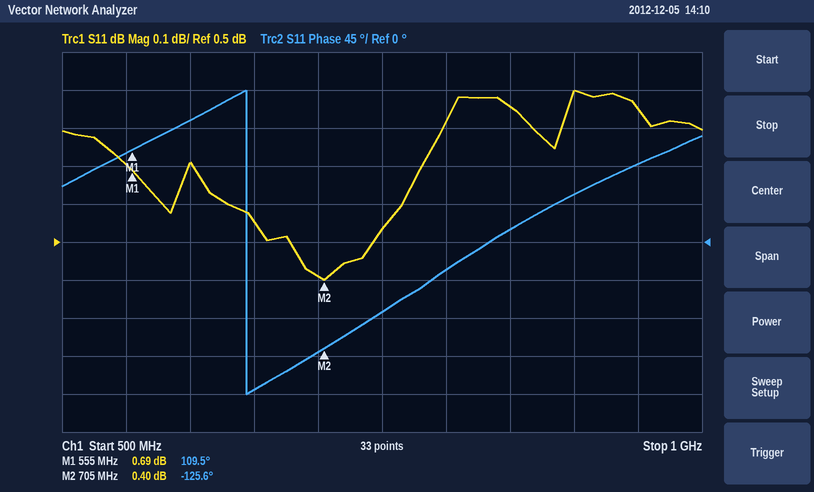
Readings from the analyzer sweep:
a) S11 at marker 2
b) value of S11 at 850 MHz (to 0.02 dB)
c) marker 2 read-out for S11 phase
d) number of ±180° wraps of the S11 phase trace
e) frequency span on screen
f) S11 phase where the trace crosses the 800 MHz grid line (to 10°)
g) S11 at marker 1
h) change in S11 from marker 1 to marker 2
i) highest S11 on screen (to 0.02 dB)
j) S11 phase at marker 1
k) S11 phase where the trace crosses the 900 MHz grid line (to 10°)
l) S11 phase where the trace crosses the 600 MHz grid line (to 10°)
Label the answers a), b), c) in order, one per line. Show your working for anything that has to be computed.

a) 0.40 dB
b) 0.86 dB
c) -125.6°
d) 1
e) 500 MHz
f) -30°
g) 0.69 dB
h) 0.4 − (0.69) = -0.29 dB
i) 0.90 dB
j) 109.5°
k) 60°
l) 140°
